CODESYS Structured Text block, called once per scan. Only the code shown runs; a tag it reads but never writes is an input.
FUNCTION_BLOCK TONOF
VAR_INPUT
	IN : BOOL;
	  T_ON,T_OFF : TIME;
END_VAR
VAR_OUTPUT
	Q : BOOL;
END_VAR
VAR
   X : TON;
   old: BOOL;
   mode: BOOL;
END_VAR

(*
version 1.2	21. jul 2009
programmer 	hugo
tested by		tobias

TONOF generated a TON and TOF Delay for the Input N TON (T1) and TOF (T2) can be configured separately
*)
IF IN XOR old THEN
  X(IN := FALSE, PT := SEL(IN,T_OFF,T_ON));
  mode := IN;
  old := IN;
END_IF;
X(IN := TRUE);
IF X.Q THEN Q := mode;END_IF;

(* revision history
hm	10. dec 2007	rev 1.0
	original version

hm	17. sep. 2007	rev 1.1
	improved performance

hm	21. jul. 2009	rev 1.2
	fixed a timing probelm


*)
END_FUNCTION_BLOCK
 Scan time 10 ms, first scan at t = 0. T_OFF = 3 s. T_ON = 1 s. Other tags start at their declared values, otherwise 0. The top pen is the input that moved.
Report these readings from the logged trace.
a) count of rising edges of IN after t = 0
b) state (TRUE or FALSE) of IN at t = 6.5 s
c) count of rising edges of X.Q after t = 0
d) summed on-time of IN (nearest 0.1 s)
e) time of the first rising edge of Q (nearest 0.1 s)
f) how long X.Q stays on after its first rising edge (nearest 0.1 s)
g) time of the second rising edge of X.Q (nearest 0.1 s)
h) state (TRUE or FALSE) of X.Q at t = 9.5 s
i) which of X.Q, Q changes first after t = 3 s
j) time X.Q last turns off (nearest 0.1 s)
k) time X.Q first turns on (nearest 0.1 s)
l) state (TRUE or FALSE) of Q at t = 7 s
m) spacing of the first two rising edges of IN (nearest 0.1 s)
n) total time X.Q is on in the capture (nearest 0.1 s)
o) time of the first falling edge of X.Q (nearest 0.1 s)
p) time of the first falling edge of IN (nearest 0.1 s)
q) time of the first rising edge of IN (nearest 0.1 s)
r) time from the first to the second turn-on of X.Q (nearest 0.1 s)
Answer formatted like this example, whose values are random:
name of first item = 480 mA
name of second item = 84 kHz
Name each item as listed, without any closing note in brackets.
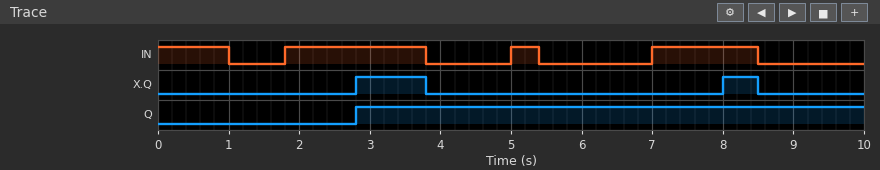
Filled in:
count of rising edges of IN after t = 0 = 3
state (TRUE or FALSE) of IN at t = 6.5 s = FALSE
count of rising edges of X.Q after t = 0 = 2
summed on-time of IN = 4.9 s
time of the first rising edge of Q = 2.8 s
how long X.Q stays on after its first rising edge = 1.0 s
time of the second rising edge of X.Q = 8.0 s
state (TRUE or FALSE) of X.Q at t = 9.5 s = FALSE
which of X.Q, Q changes first after t = 3 s = X.Q
time X.Q last turns off = 8.5 s
time X.Q first turns on = 2.8 s
state (TRUE or FALSE) of Q at t = 7 s = TRUE
spacing of the first two rising edges of IN = 3.2 s
total time X.Q is on in the capture = 1.5 s
time of the first falling edge of X.Q = 3.8 s
time of the first falling edge of IN = 1.0 s
time of the first rising edge of IN = 1.8 s
time from the first to the second turn-on of X.Q = 5.2 s
